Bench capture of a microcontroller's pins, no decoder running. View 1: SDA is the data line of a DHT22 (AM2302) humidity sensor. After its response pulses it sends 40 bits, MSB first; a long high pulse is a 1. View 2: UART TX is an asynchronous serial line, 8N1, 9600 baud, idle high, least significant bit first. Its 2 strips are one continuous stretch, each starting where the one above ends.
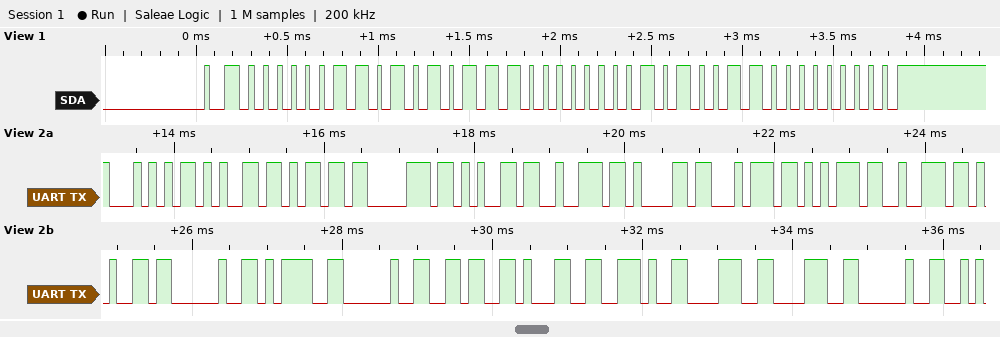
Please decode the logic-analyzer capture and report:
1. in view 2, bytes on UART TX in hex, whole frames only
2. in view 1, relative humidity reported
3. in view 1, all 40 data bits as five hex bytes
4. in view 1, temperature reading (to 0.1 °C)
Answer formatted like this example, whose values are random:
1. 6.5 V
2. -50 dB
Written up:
1. 54 65 6D 70 65 72 61 74 75 72 65 20 3D 20 36 31 2E 38 38 20
2. 85.5 %
3. 03 57 00 A6 00
4. 16.6 °C
